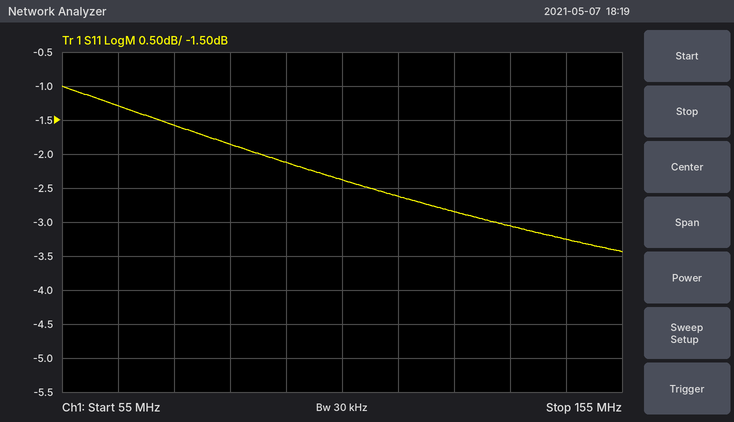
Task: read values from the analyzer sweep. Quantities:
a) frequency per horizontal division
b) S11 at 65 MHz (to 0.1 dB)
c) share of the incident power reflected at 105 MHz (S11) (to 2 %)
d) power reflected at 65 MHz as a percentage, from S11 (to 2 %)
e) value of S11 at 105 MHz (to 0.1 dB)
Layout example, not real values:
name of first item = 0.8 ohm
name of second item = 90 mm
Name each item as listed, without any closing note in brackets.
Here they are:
frequency per horizontal division = 10 MHz
S11 at 65 MHz = -1.3 dB
share of the incident power reflected at 105 MHz (S11) = 58 %
power reflected at 65 MHz as a percentage, from S11 = 74 %
value of S11 at 105 MHz = -2.4 dB
